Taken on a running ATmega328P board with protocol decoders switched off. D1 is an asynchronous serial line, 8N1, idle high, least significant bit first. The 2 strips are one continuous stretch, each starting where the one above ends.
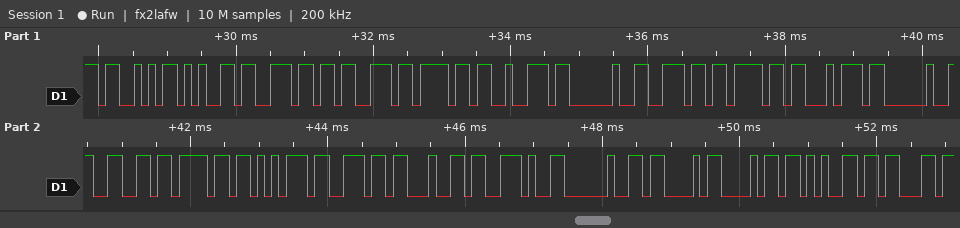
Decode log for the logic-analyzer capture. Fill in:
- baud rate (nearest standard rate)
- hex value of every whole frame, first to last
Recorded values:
9600 baud
0x53 0x65 0x6E 0x73 0x6F 0x72 0x20 0x6E 0x6F 0x74 0x20 0x66 0x6F 0x75 0x6E 0x64 0x2E 0x20 0x43 0x68 0x65 0x63
